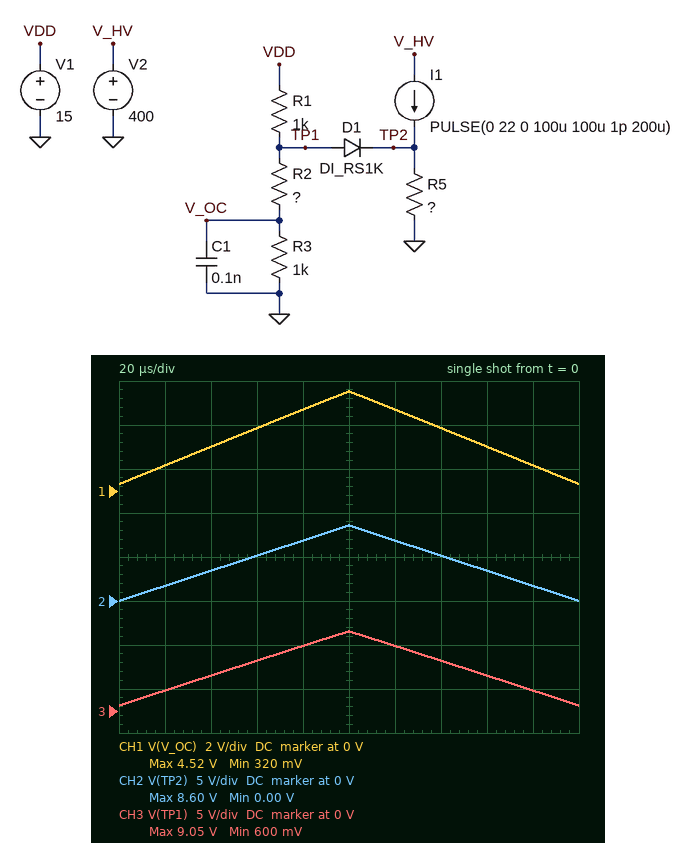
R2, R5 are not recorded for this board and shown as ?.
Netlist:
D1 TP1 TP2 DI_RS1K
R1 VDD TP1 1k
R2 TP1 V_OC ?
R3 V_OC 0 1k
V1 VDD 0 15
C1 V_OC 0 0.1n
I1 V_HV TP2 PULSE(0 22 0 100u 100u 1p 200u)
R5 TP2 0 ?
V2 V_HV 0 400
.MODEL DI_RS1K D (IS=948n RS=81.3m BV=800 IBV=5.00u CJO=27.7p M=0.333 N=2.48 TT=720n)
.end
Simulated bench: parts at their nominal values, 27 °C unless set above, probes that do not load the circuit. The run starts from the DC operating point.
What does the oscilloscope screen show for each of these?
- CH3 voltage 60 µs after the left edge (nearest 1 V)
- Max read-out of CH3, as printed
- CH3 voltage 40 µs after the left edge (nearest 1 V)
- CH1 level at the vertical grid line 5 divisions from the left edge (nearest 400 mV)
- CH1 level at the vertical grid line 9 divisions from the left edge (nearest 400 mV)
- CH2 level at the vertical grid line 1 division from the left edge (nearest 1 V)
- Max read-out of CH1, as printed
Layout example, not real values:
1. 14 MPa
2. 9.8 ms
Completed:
1. 6 V
2. 9.05 V
3. 4 V
4. 4.4 V
5. 1.2 V
6. 2 V
7. 4.52 V
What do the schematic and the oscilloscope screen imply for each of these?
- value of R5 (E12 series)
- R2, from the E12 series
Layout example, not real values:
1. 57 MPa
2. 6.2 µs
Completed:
1. 0.39 Ω
2. 1 kΩ
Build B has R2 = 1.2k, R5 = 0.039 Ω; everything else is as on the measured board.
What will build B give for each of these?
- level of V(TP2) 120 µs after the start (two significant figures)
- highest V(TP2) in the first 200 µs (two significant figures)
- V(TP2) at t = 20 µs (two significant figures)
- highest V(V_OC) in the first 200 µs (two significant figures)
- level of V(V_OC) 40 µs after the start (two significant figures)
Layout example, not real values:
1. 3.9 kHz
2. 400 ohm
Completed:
1. 690 mV
2. 860 mV
3. 170 mV
4. 670 mV
5. 440 mV
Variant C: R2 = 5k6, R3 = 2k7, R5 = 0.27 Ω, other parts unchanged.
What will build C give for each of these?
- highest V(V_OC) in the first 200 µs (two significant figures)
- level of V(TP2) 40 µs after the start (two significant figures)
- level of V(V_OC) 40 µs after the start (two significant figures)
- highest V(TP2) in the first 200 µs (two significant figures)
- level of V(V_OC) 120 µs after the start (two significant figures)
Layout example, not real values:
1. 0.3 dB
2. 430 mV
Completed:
1. 2.1 V
2. 2.4 V
3. 970 mV
4. 5.9 V
5. 1.7 V
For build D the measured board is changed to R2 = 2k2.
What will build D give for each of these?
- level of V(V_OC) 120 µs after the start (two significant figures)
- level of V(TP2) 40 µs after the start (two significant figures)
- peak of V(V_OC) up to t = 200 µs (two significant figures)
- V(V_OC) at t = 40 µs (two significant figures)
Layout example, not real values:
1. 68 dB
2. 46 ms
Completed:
1. 2.3 V
2. 3.4 V
3. 2.8 V
4. 1.3 V
